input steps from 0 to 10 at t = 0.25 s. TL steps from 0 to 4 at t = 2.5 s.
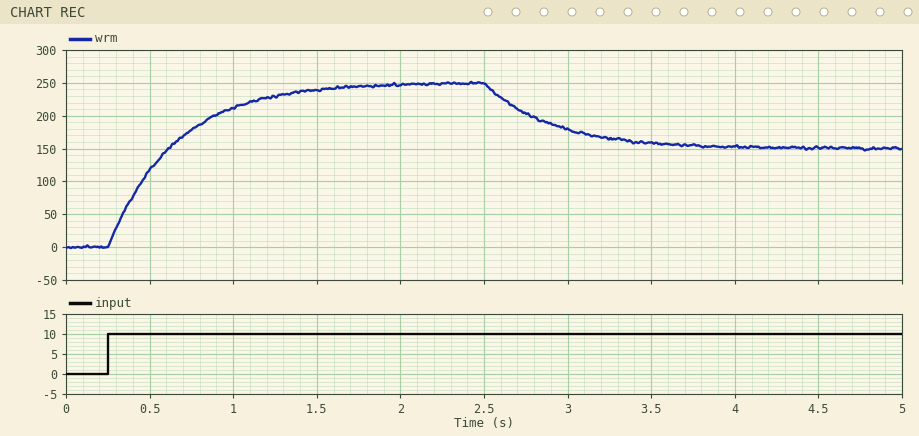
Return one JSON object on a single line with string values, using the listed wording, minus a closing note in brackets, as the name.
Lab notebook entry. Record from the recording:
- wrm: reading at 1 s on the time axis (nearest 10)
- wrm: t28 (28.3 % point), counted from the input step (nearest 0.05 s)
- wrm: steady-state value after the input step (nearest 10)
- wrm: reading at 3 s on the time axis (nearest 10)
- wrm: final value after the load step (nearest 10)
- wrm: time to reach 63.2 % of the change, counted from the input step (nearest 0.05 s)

{"wrm: reading at 1 s on the time axis": "210", "wrm: t28 (28.3 % point), counted from the input step": "0.15 s", "wrm: steady-state value after the input step": "250", "wrm: reading at 3 s on the time axis": "180", "wrm: final value after the load step": "150", "wrm: time to reach 63.2 % of the change, counted from the input step": "0.40 s"}
